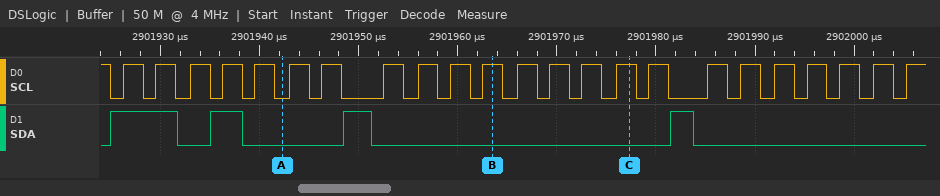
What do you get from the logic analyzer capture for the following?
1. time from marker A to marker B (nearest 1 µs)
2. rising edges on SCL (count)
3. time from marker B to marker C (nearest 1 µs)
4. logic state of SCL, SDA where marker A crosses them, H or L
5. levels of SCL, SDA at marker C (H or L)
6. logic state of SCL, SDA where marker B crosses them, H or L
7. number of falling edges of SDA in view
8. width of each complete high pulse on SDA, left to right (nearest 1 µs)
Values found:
21 µs
23
14 µs
SCL=L, SDA=L
SCL=H, SDA=L
SCL=H, SDA=L
4
7 µs, 3 µs, 3 µs, 2 µs
